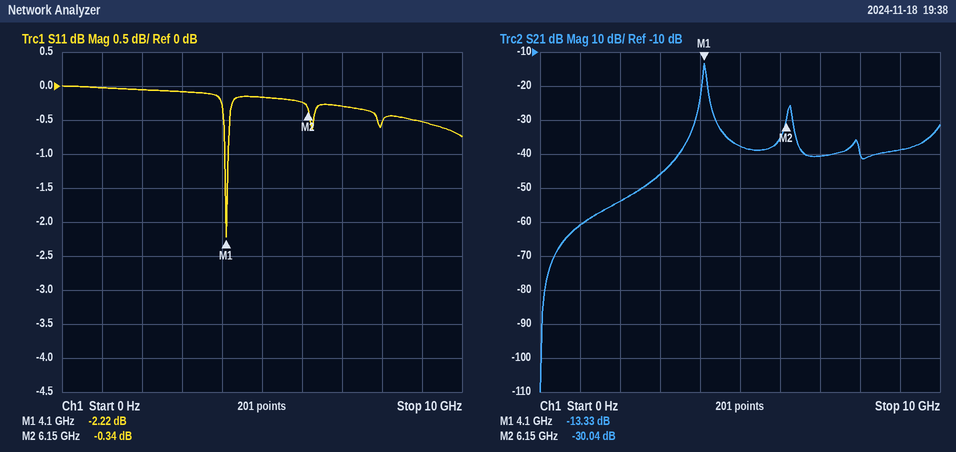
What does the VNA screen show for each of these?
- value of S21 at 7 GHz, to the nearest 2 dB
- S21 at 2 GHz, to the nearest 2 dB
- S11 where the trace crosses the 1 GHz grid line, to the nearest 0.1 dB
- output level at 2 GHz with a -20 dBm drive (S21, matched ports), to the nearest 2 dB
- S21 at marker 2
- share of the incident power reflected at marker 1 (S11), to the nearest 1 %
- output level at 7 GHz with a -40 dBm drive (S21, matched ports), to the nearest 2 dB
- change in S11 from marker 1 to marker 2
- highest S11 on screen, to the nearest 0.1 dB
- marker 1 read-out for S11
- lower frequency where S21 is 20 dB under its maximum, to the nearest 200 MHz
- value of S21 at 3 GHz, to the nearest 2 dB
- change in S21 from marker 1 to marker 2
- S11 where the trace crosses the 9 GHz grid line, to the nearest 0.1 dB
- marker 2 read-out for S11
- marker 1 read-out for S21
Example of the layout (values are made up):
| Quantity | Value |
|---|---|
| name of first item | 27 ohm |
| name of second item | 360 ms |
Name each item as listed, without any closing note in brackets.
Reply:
| Quantity | Value |
|---|---|
| value of S21 at 7 GHz, to the nearest 2 dB | -40 dB |
| S21 at 2 GHz, to the nearest 2 dB | -54 dB |
| S11 where the trace crosses the 1 GHz grid line, to the nearest 0.1 dB | 0.0 dB |
| output level at 2 GHz with a -20 dBm drive (S21, matched ports), to the nearest 2 dB | -74 dBm |
| S21 at marker 2 | -30.04 dB |
| share of the incident power reflected at marker 1 (S11), to the nearest 1 % | 60 % |
| output level at 7 GHz with a -40 dBm drive (S21, matched ports), to the nearest 2 dB | -80 dBm |
| change in S11 from marker 1 to marker 2 | 1.88 dB |
| highest S11 on screen, to the nearest 0.1 dB | 0.0 dB |
| marker 1 read-out for S11 | -2.22 dB |
| lower frequency where S21 is 20 dB under its maximum, to the nearest 200 MHz | 3.8 GHz |
| value of S21 at 3 GHz, to the nearest 2 dB | -46 dB |
| change in S21 from marker 1 to marker 2 | -16.71 dB |
| S11 where the trace crosses the 9 GHz grid line, to the nearest 0.1 dB | -0.5 dB |
| marker 2 read-out for S11 | -0.34 dB |
| marker 1 read-out for S21 | -13.33 dB |
